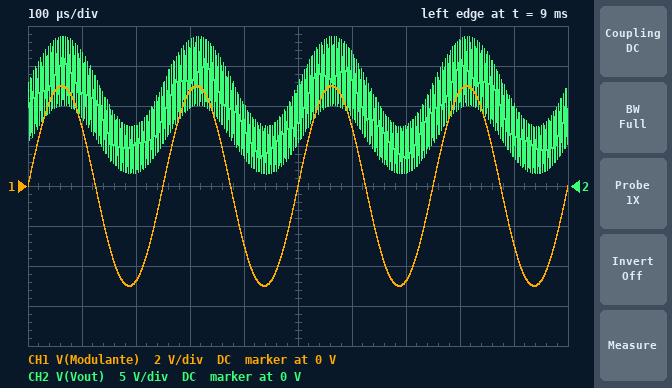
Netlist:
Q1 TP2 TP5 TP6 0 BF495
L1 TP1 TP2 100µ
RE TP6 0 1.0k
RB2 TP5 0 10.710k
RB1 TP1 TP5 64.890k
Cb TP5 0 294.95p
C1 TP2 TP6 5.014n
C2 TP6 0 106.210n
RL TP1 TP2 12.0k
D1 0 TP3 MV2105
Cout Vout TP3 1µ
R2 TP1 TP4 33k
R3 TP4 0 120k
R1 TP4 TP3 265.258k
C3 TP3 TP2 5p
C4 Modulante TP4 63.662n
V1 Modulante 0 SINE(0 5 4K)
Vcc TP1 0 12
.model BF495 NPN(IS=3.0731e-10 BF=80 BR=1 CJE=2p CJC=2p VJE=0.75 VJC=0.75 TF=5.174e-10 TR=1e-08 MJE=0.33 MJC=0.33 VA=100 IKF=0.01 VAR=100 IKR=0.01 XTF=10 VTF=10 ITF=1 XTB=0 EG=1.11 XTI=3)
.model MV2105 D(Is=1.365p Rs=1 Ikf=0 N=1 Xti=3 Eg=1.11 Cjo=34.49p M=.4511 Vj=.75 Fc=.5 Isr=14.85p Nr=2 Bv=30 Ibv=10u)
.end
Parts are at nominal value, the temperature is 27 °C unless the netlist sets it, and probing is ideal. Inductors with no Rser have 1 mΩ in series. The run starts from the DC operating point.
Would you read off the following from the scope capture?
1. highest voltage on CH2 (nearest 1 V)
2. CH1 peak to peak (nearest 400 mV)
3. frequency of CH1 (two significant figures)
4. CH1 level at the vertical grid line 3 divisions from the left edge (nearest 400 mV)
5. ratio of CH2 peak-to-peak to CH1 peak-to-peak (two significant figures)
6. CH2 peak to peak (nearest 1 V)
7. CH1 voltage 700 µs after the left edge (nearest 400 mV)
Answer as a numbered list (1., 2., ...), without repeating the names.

1. 19 V
2. 10.0 V
3. 4.0 kHz
4. 4.8 V
5. 1.7
6. 17 V
7. -4.8 V
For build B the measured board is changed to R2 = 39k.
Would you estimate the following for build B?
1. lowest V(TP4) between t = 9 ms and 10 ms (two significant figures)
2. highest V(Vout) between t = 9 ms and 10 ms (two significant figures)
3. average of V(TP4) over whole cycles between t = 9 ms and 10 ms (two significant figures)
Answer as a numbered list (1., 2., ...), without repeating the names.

1. 4.0 V
2. 18 V
3. 9.0 V
